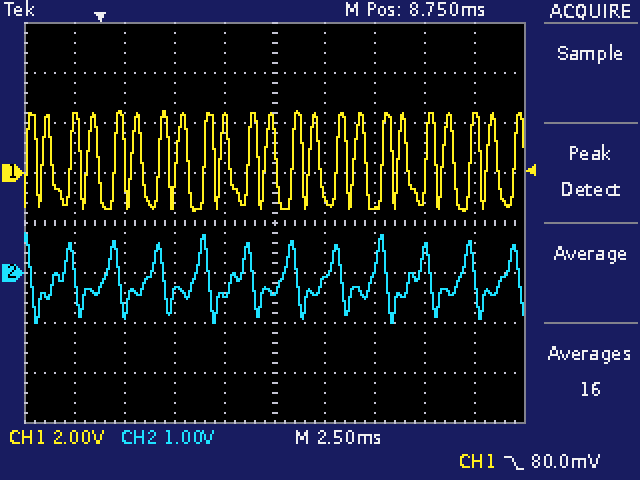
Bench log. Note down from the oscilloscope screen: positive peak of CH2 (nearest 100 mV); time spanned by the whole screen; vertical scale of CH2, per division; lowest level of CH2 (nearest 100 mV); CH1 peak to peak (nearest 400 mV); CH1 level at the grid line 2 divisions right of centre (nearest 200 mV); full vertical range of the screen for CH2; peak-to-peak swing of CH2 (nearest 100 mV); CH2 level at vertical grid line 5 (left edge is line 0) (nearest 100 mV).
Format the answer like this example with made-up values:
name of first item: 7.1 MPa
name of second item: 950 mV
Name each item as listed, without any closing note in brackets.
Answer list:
positive peak of CH2: 800 mV
time spanned by the whole screen: 25 ms
vertical scale of CH2, per division: 1 V
lowest level of CH2: -1.0 V
CH1 peak to peak: 4.0 V
CH1 level at the grid line 2 divisions right of centre: -1.4 V
full vertical range of the screen for CH2: 8 V
peak-to-peak swing of CH2: 1.8 V
CH2 level at vertical grid line 5 (left edge is line 0): -400 mV
